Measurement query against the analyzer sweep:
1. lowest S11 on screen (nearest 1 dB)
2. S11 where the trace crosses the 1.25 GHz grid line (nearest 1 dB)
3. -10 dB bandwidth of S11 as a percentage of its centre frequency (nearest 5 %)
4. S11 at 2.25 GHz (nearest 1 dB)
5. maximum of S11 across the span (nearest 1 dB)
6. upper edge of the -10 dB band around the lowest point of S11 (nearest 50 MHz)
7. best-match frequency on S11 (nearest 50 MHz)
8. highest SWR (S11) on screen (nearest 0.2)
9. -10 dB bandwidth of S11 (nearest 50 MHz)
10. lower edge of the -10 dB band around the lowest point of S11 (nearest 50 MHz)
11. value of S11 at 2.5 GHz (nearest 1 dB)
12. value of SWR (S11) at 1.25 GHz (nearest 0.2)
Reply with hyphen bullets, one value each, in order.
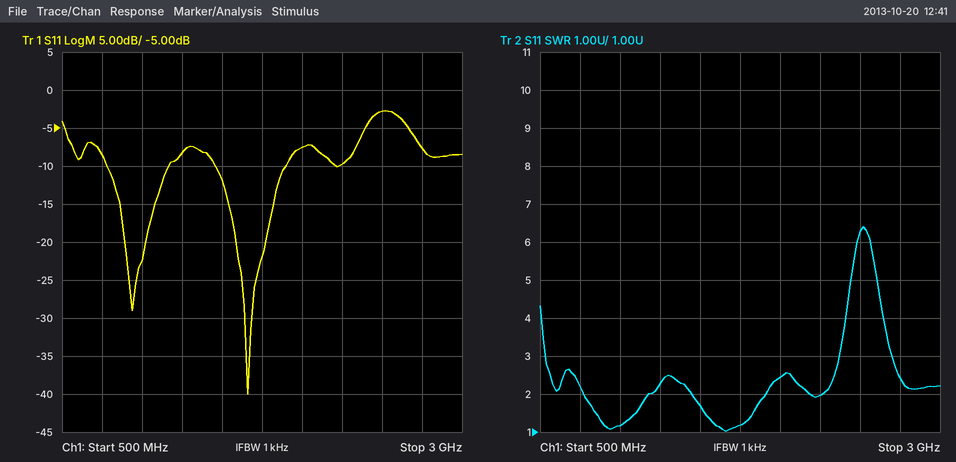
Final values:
- -40 dB
- -8 dB
- 25 %
- -10 dB
- -3 dB
- 1.90 GHz
- 1.65 GHz
- 6.4
- 450 MHz
- 1.45 GHz
- -3 dB
- 2.2
